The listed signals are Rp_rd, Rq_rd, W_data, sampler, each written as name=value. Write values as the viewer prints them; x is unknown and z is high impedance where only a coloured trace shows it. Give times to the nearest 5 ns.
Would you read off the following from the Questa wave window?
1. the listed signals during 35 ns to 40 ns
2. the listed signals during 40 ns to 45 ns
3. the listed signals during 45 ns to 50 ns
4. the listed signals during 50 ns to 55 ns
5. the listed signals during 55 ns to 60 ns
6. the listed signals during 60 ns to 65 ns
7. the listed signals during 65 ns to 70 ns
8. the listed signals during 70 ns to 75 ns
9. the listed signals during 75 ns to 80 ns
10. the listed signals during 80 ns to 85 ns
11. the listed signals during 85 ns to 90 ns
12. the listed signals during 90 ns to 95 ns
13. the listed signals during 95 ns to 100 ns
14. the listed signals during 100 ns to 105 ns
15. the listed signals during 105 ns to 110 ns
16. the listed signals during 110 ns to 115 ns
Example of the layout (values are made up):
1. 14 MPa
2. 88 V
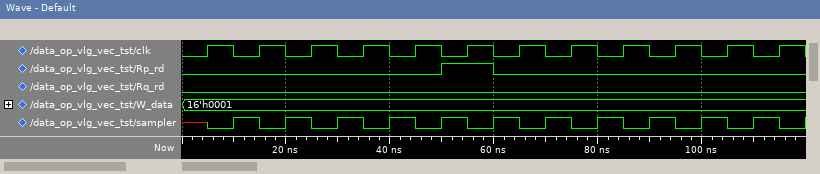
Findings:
1. Rp_rd=0, Rq_rd=0, W_data=16'h0001, sampler=0
2. Rp_rd=0, Rq_rd=0, W_data=16'h0001, sampler=1
3. Rp_rd=0, Rq_rd=0, W_data=16'h0001, sampler=0
4. Rp_rd=1, Rq_rd=0, W_data=16'h0001, sampler=1
5. Rp_rd=1, Rq_rd=0, W_data=16'h0001, sampler=0
6. Rp_rd=0, Rq_rd=0, W_data=16'h0001, sampler=1
7. Rp_rd=0, Rq_rd=0, W_data=16'h0001, sampler=0
8. Rp_rd=0, Rq_rd=0, W_data=16'h0001, sampler=1
9. Rp_rd=0, Rq_rd=0, W_data=16'h0001, sampler=0
10. Rp_rd=0, Rq_rd=0, W_data=16'h0001, sampler=1
11. Rp_rd=0, Rq_rd=0, W_data=16'h0001, sampler=0
12. Rp_rd=0, Rq_rd=0, W_data=16'h0001, sampler=1
13. Rp_rd=0, Rq_rd=0, W_data=16'h0001, sampler=0
14. Rp_rd=0, Rq_rd=0, W_data=16'h0001, sampler=1
15. Rp_rd=0, Rq_rd=0, W_data=16'h0001, sampler=0
16. Rp_rd=0, Rq_rd=0, W_data=16'h0001, sampler=1
